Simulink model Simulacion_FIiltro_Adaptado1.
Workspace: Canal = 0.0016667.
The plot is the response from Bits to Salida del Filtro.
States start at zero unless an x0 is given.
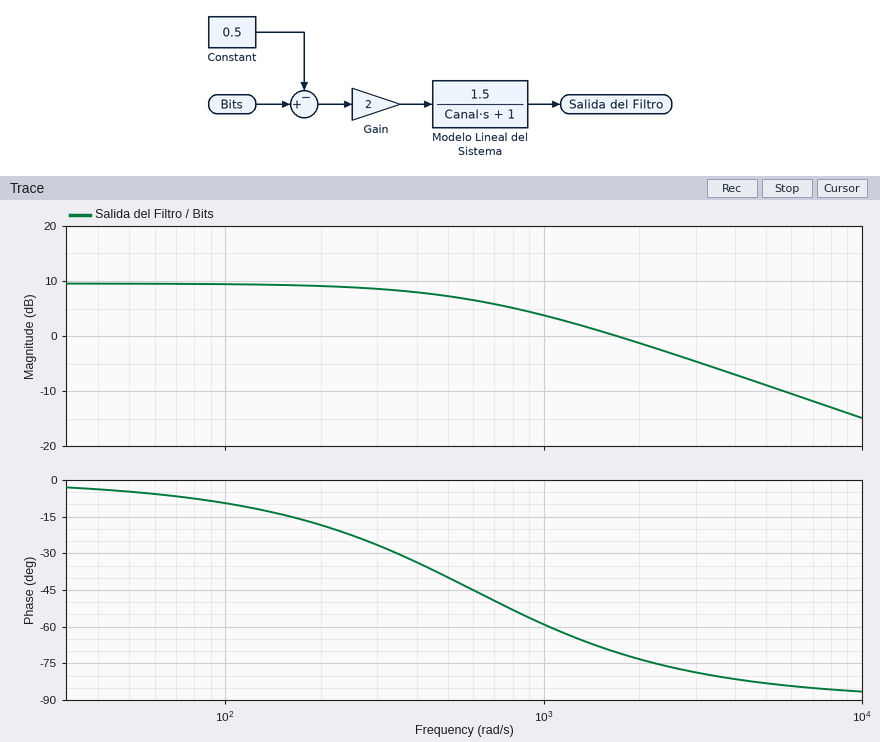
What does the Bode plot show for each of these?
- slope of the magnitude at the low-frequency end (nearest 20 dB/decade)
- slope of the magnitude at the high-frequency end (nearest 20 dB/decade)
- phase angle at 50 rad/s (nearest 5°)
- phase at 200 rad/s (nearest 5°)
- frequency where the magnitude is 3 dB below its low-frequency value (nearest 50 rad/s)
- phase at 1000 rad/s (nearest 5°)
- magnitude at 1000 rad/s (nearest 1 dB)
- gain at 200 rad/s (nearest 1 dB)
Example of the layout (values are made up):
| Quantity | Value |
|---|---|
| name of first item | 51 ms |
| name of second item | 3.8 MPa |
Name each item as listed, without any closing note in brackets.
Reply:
| Quantity | Value |
|---|---|
| slope of the magnitude at the low-frequency end | 0 dB/decade |
| slope of the magnitude at the high-frequency end | -20 dB/decade |
| phase angle at 50 rad/s | -5° |
| phase at 200 rad/s | -20° |
| frequency where the magnitude is 3 dB below its low-frequency value | 600 rad/s |
| phase at 1000 rad/s | -60° |
| magnitude at 1000 rad/s | 4 dB |
| gain at 200 rad/s | 9 dB |
